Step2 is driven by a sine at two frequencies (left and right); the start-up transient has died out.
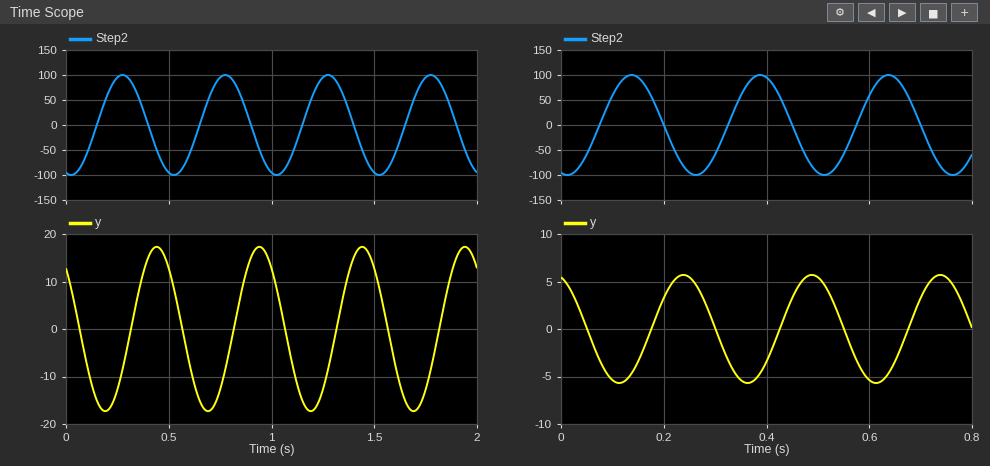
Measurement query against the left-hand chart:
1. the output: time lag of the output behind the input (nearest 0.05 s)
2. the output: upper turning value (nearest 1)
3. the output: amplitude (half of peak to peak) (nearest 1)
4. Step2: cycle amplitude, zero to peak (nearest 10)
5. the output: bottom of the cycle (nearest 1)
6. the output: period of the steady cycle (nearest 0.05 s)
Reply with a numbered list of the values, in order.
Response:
1. 0.15 s
2. 17
3. 17
4. 100
5. -17
6. 0.50 s
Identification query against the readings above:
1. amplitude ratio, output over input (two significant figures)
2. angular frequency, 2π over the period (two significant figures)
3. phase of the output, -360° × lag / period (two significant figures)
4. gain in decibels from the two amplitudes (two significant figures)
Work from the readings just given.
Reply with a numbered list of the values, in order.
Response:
1. 0.17
2. 13 rad/s
3. -110°
4. -15 dB
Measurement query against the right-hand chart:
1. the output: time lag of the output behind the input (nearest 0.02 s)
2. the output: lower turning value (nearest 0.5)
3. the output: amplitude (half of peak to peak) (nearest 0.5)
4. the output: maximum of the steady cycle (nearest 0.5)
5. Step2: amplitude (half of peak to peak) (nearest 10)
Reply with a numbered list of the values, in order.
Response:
1. 0.10 s
2. -5.5
3. 5.5
4. 5.5
5. 100
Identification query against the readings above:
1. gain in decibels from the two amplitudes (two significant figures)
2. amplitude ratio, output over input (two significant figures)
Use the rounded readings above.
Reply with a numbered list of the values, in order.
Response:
1. -25 dB
2. 0.055
